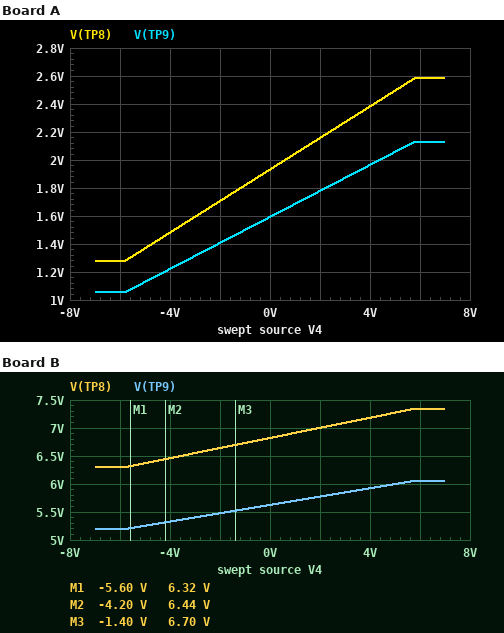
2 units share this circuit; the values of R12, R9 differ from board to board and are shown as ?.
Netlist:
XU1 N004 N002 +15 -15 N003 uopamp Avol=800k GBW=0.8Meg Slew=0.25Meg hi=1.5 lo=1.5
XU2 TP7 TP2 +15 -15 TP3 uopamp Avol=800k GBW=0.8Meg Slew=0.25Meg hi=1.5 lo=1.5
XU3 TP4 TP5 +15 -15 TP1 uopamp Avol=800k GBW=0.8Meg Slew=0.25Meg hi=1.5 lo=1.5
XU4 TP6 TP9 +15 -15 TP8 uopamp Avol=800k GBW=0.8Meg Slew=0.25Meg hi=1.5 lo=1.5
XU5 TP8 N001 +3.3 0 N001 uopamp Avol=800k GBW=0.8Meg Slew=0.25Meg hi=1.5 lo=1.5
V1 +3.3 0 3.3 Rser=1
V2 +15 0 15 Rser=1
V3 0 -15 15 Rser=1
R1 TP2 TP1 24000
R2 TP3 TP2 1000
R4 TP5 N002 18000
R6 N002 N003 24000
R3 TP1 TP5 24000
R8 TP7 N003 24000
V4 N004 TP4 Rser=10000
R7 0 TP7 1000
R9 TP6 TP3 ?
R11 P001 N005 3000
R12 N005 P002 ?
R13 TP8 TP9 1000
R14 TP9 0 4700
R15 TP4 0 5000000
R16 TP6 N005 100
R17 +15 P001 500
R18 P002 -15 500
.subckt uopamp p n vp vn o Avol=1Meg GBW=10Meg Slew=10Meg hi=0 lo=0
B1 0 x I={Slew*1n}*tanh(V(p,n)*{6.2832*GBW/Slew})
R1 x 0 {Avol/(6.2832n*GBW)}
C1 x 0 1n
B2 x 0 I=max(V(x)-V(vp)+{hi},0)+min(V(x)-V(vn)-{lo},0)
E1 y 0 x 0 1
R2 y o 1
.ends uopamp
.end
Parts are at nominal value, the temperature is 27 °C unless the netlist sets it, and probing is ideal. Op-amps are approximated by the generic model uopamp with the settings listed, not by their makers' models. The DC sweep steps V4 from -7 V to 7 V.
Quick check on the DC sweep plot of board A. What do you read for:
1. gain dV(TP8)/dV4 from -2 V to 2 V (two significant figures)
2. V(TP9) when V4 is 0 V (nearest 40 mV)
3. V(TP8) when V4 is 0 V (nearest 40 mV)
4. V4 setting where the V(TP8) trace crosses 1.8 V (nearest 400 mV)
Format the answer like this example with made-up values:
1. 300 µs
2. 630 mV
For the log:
1. 0.11 V/V
2. 1.60 V
3. 1.92 V
4. -1.2 V
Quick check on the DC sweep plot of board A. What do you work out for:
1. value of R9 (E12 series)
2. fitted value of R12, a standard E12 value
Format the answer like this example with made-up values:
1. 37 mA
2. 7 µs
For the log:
1. 1.5 kΩ
2. 5.6 kΩ
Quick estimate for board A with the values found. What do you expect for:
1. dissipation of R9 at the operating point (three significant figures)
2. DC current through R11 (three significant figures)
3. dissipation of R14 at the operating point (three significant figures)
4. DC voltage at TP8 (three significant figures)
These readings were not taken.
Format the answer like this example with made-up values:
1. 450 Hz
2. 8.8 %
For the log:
1. 1.69 mW
2. 3.80 mA
3. 540 µW
4. 1.93 V
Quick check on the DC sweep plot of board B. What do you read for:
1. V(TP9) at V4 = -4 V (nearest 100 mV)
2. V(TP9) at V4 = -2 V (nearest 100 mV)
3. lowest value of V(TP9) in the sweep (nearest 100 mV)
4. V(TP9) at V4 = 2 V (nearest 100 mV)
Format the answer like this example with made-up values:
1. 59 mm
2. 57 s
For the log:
1. 5.3 V
2. 5.5 V
3. 5.2 V
4. 5.8 V
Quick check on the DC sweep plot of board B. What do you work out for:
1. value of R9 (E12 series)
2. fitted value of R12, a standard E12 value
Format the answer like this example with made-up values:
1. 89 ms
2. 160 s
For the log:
1. 3.3 kΩ
2. 22 kΩ
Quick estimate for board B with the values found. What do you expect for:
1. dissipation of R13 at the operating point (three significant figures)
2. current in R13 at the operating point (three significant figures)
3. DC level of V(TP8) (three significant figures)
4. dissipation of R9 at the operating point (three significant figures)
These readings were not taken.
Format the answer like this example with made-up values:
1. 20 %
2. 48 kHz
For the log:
1. 1.43 mW
2. 1.20 mA
3. 6.82 V
4. 9.59 mW
